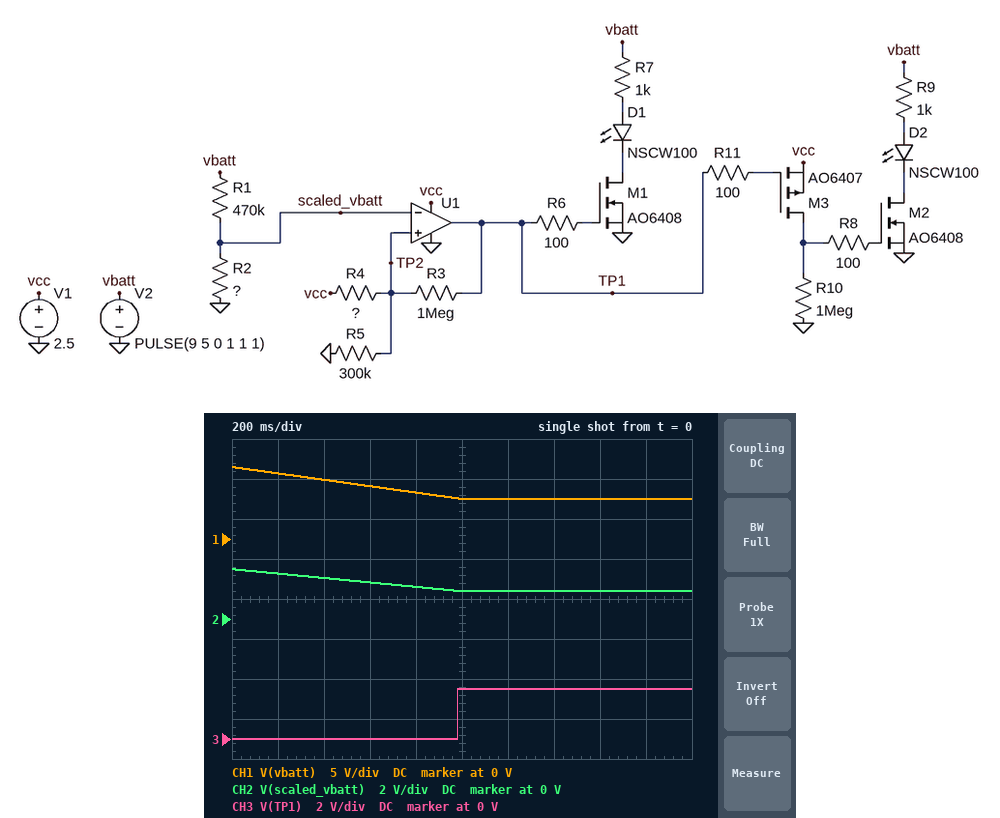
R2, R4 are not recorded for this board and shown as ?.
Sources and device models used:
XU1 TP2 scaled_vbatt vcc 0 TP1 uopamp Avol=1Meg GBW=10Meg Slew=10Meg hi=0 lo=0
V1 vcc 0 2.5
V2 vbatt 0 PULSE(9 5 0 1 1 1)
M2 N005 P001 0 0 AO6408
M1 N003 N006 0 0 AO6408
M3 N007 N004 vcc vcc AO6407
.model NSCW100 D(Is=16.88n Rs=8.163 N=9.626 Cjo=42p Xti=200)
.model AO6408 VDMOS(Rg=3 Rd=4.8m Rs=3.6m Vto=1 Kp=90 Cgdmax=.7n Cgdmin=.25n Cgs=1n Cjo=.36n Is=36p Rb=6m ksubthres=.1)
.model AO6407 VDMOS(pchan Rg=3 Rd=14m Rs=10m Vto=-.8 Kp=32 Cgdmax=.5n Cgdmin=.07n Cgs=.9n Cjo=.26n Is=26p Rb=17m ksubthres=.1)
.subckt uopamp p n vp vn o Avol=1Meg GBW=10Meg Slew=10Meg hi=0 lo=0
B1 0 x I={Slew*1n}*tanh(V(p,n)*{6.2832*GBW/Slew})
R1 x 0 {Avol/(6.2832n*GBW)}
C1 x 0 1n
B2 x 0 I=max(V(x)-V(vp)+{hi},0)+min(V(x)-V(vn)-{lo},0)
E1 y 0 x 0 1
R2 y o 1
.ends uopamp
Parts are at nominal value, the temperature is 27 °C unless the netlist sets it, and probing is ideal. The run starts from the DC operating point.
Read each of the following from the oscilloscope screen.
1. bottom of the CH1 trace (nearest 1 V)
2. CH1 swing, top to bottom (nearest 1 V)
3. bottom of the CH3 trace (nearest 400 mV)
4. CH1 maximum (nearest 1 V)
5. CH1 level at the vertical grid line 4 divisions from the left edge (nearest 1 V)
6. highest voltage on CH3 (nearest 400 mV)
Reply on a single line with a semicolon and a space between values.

5 V; 4 V; 0 V; 9 V; 6 V; 2.4 V
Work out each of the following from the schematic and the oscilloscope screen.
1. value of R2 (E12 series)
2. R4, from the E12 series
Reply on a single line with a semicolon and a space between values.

180 kΩ; 180 kΩ
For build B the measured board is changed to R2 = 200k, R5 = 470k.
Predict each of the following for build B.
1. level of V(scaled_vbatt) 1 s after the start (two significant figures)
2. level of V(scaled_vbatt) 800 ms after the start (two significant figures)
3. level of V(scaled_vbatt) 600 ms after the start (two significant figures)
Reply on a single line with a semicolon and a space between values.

1.5 V; 1.7 V; 2.0 V
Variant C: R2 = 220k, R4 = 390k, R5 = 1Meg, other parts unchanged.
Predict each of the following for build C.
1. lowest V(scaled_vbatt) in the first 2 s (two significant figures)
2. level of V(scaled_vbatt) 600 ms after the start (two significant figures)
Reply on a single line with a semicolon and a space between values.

1.6 V; 2.1 V
